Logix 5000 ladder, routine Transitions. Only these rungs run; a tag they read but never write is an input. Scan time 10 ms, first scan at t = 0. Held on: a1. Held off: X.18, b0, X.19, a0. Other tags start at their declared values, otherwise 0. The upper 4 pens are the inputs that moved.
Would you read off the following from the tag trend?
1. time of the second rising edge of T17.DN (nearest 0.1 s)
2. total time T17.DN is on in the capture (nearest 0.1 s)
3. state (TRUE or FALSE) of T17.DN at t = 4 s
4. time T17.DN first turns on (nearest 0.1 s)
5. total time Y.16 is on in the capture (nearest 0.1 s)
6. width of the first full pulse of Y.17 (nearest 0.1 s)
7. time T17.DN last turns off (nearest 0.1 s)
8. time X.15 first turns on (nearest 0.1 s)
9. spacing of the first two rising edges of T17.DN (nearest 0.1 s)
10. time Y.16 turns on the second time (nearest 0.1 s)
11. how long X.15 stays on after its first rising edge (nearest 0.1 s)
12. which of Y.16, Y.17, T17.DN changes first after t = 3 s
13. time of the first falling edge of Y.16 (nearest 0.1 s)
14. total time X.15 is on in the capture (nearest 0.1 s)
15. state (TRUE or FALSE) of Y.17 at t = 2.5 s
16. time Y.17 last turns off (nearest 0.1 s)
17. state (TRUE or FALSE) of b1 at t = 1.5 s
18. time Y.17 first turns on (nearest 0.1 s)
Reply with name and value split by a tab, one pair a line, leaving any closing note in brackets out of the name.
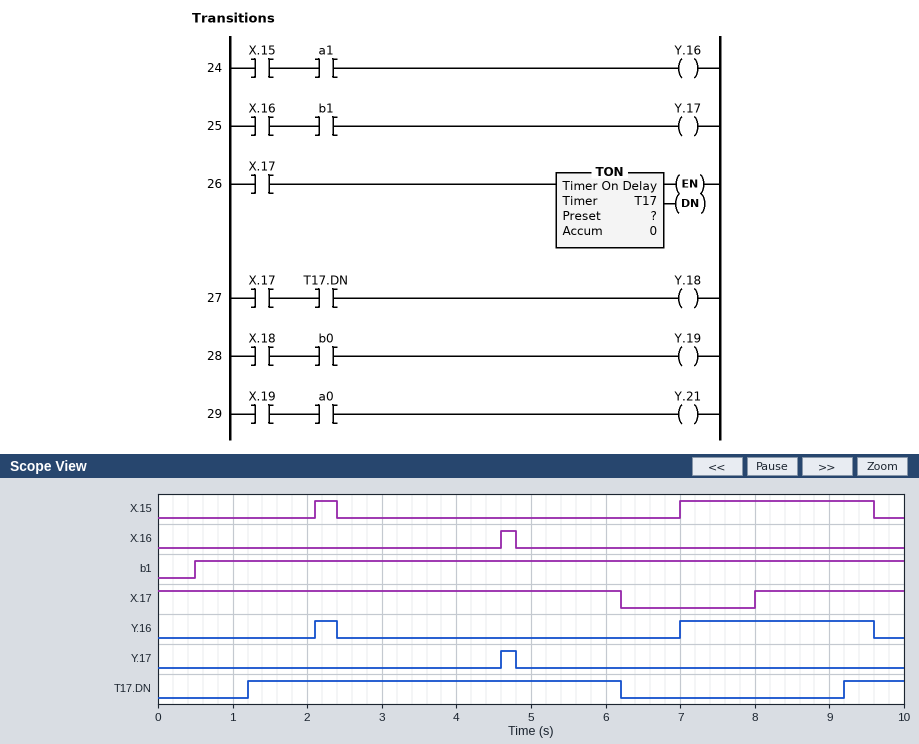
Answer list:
time of the second rising edge of T17.DN	9.2 s
total time T17.DN is on in the capture	5.8 s
state (TRUE or FALSE) of T17.DN at t = 4 s	TRUE
time T17.DN first turns on	1.2 s
total time Y.16 is on in the capture	2.9 s
width of the first full pulse of Y.17	0.2 s
time T17.DN last turns off	6.2 s
time X.15 first turns on	2.1 s
spacing of the first two rising edges of T17.DN	8.0 s
time Y.16 turns on the second time	7.0 s
how long X.15 stays on after its first rising edge	0.3 s
which of Y.16, Y.17, T17.DN changes first after t = 3 s	Y.17
time of the first falling edge of Y.16	2.4 s
total time X.15 is on in the capture	2.9 s
state (TRUE or FALSE) of Y.17 at t = 2.5 s	FALSE
time Y.17 last turns off	4.8 s
state (TRUE or FALSE) of b1 at t = 1.5 s	TRUE
time Y.17 first turns on	4.6 s
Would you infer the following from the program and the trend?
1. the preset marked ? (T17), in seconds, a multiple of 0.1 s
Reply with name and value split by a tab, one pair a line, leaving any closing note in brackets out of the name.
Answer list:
the preset marked ? (T17), in seconds, a multiple of 0.1 s	1.2 s
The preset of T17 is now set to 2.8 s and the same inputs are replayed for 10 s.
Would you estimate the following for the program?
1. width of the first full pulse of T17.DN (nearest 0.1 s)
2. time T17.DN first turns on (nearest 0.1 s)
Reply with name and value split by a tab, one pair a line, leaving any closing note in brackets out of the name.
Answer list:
width of the first full pulse of T17.DN	3.4 s
time T17.DN first turns on	2.8 s
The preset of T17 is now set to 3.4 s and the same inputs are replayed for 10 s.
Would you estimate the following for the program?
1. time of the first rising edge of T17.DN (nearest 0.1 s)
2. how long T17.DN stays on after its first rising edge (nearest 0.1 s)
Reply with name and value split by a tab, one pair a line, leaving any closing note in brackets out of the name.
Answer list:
time of the first rising edge of T17.DN	3.4 s
how long T17.DN stays on after its first rising edge	2.8 s
